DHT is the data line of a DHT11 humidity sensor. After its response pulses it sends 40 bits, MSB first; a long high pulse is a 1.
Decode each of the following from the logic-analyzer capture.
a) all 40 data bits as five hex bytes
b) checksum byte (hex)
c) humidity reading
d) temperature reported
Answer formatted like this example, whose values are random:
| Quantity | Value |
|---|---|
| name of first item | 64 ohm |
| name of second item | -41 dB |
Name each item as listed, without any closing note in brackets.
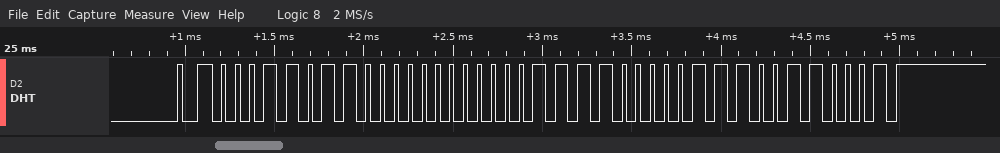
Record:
| Quantity | Value |
|---|---|
| all 40 data bits as five hex bytes | 1B 00 0F 07 31 |
| checksum byte | 0x31 |
| humidity reading | 27 % |
| temperature reported | 15.7 °C |
